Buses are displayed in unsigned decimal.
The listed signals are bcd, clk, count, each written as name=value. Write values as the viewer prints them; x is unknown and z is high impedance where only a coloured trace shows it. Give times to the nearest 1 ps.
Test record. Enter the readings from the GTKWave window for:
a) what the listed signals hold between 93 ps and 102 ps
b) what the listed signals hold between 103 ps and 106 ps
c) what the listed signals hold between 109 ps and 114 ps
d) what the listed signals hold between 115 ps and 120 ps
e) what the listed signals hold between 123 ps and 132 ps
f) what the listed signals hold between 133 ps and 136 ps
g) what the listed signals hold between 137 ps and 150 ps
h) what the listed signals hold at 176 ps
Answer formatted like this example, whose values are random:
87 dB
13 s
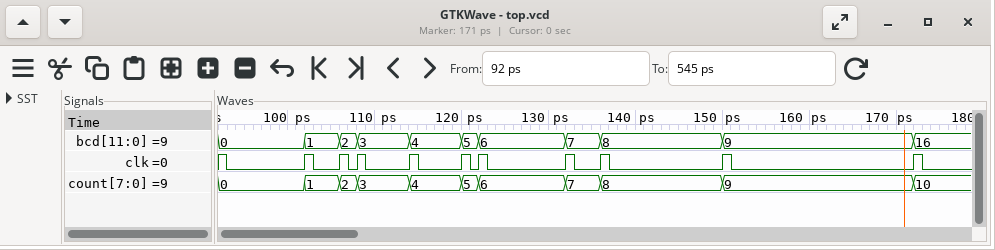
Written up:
bcd=0, clk=0, count=0
bcd=1, clk=0, count=1
bcd=3, clk=0, count=3
bcd=4, clk=0, count=4
bcd=6, clk=0, count=6
bcd=7, clk=0, count=7
bcd=8, clk=0, count=8
bcd=16, clk=0, count=10
